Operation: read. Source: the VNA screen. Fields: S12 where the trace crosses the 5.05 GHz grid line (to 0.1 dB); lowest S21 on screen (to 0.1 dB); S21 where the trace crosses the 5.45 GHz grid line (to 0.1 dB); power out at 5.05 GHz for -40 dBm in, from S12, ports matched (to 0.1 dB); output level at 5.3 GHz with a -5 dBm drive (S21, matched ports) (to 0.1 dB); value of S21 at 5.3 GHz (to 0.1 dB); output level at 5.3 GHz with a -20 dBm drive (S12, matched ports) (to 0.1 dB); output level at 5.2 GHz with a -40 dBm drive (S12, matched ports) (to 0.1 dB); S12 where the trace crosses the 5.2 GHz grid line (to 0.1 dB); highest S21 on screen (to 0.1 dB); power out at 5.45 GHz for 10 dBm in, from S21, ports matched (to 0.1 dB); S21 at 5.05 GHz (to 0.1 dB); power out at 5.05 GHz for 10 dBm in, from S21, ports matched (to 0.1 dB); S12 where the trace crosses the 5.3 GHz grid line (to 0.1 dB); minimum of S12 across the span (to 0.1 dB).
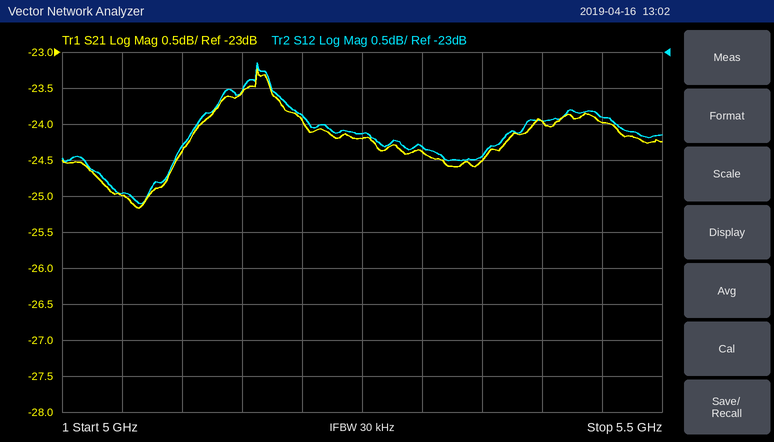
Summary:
-25.0 dB
-25.2 dB
-24.0 dB
-65.0 dBm
-29.4 dBm
-24.4 dB
-44.3 dBm
-63.9 dBm
-23.9 dB
-23.2 dB
-14.0 dBm
-25.0 dB
-15.0 dBm
-24.3 dB
-25.1 dB
